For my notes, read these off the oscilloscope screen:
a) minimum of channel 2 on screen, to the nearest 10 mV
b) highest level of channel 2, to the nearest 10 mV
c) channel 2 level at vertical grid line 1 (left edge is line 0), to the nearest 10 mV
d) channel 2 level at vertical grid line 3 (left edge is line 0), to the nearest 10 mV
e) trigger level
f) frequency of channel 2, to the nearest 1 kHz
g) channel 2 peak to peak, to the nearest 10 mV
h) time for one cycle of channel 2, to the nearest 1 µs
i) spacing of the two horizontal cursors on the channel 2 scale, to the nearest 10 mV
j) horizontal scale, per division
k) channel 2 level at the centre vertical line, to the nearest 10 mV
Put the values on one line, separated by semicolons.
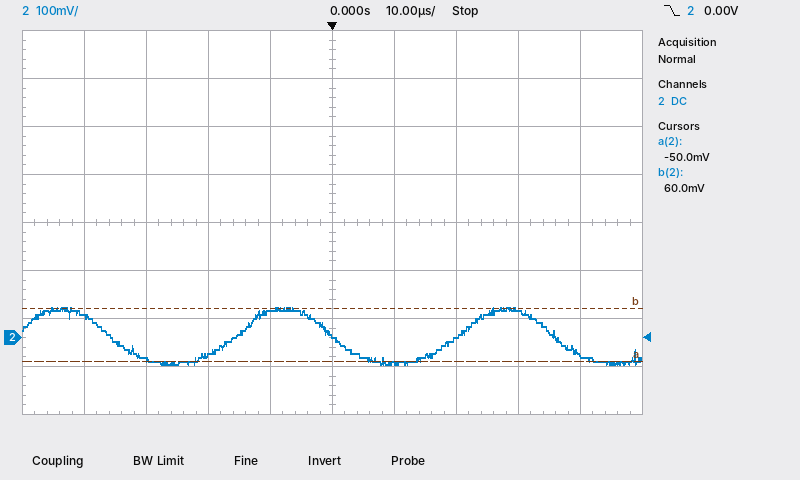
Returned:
-60 mV; 60 mV; 40 mV; -40 mV; 0.00 V; 28 kHz; 120 mV; 36 µs; 110 mV; 10 µs; 10 mV
